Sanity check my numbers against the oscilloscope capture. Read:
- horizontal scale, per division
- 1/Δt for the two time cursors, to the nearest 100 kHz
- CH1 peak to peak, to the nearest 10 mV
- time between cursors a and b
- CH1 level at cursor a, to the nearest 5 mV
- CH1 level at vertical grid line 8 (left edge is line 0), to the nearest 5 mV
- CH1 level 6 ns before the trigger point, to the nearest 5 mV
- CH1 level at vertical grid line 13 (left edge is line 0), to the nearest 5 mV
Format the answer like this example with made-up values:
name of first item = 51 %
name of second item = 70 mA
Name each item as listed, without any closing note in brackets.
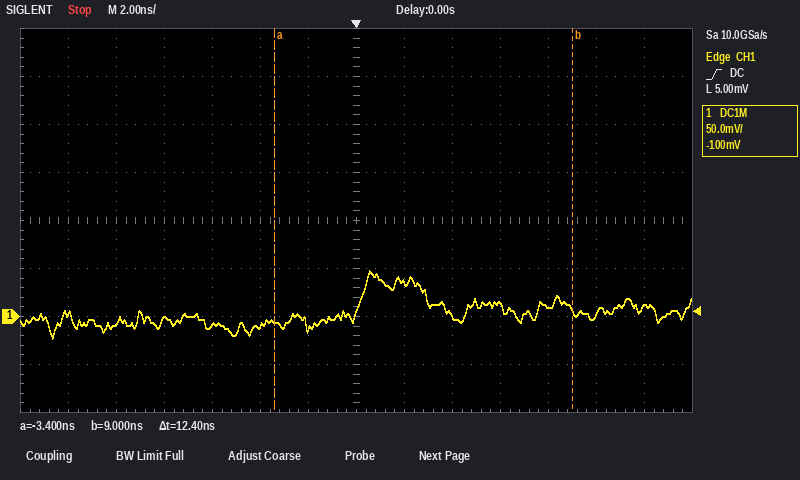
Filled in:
horizontal scale, per division = 2 ns
1/Δt for the two time cursors, to the nearest 100 kHz = 80.6 MHz
CH1 peak to peak, to the nearest 10 mV = 70 mV
time between cursors a and b = 12.4 ns
CH1 level at cursor a, to the nearest 5 mV = -5 mV
CH1 level at vertical grid line 8 (left edge is line 0), to the nearest 5 mV = 35 mV
CH1 level 6 ns before the trigger point, to the nearest 5 mV = -10 mV
CH1 level at vertical grid line 13 (left edge is line 0), to the nearest 5 mV = 10 mV
